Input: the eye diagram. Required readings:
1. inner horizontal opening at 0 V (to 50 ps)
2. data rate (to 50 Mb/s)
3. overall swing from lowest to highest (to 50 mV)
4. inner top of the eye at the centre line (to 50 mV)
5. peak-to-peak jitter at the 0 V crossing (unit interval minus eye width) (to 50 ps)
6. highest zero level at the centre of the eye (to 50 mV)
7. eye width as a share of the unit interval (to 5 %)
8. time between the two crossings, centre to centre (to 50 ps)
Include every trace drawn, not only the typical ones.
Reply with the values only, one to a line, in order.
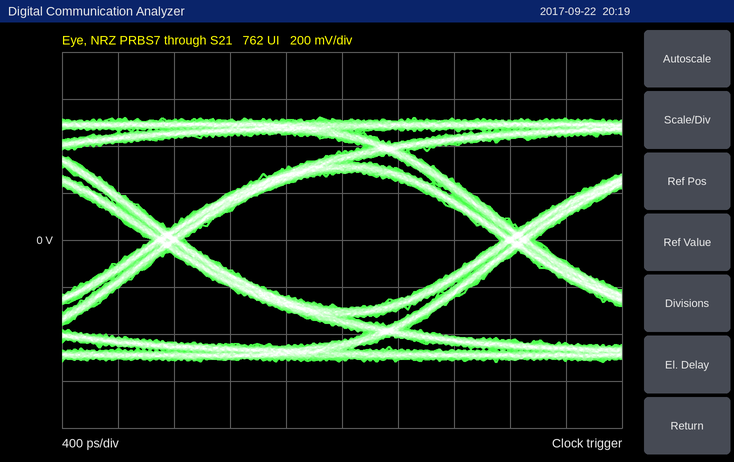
2.25 ns
400 Mb/s
1.05 V
300 mV
250 ps
-300 mV
90 %
2.50 ns
